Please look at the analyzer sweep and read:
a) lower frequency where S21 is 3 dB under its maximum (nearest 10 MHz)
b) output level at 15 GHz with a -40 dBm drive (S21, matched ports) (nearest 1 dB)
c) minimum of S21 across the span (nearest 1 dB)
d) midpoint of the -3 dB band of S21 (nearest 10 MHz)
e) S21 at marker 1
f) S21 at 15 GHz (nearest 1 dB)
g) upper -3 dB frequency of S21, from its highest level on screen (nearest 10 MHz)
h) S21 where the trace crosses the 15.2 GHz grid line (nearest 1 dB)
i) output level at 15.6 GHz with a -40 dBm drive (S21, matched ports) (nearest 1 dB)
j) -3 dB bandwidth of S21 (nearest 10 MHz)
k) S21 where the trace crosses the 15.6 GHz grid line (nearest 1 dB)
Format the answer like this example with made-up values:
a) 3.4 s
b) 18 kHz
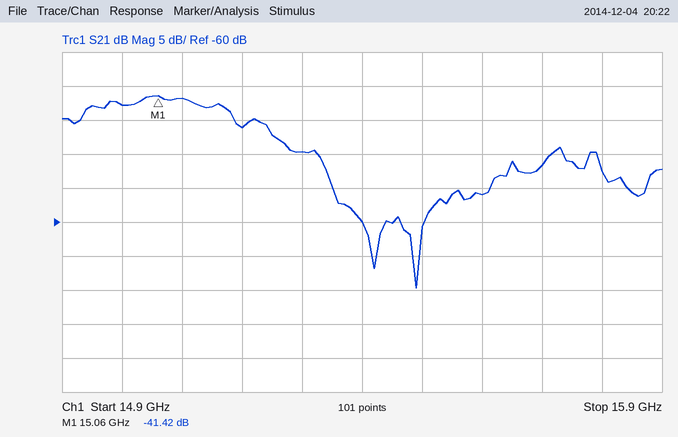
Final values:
a) 14.93 GHz
b) -83 dBm
c) -70 dB
d) 15.06 GHz
e) -41.42 dB
f) -43 dB
g) 15.18 GHz
h) -46 dB
i) -96 dBm
j) 250 MHz
k) -56 dB
